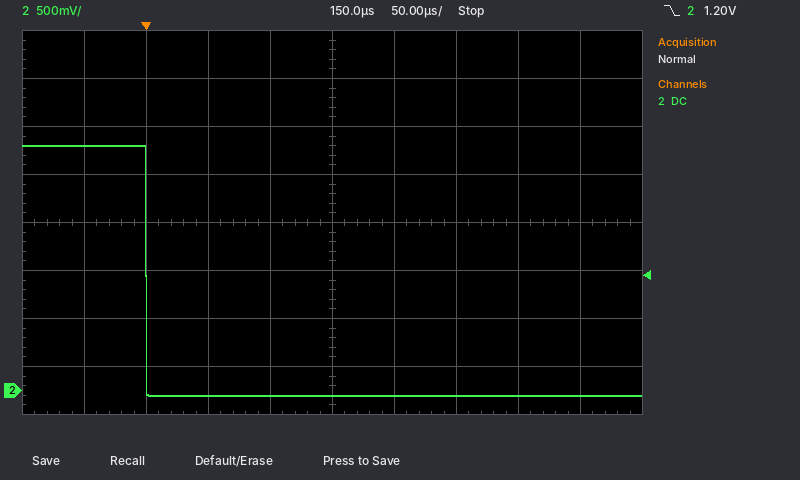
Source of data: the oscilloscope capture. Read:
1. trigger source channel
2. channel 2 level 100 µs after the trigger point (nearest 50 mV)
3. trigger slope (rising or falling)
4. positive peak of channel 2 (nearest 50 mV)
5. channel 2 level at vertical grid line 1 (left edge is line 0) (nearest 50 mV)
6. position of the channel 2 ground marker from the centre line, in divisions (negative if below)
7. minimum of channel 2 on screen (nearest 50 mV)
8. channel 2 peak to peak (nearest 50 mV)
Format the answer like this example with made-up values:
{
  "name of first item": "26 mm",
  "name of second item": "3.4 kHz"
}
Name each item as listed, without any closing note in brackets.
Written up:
{
  "trigger source channel": "channel 2",
  "channel 2 level 100 µs after the trigger point": "-50 mV",
  "trigger slope": "falling",
  "positive peak of channel 2": "2.55 V",
  "channel 2 level at vertical grid line 1 (left edge is line 0)": "2.55 V",
  "position of the channel 2 ground marker from the centre line, in divisions": "-3.5 div",
  "minimum of channel 2 on screen": "-50 mV",
  "channel 2 peak to peak": "2.60 V"
}
